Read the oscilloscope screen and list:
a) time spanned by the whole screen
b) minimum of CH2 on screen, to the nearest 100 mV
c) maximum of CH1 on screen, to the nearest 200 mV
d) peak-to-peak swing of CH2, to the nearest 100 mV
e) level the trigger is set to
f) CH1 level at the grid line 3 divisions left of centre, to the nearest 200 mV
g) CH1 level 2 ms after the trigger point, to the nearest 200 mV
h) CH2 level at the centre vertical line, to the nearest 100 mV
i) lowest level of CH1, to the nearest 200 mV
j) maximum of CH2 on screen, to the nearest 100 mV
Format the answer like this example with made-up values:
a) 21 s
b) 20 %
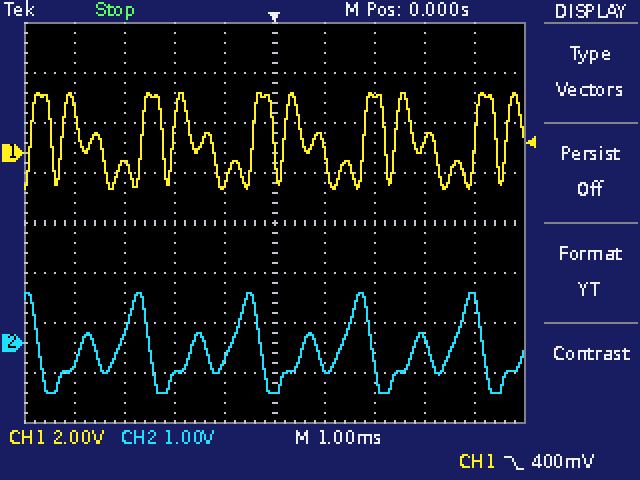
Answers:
a) 10 ms
b) -1.0 V
c) 2.4 V
d) 2.0 V
e) 400 mV
f) -400 mV
g) 2.4 V
h) -1.0 V
i) -1.4 V
j) 1.0 V
